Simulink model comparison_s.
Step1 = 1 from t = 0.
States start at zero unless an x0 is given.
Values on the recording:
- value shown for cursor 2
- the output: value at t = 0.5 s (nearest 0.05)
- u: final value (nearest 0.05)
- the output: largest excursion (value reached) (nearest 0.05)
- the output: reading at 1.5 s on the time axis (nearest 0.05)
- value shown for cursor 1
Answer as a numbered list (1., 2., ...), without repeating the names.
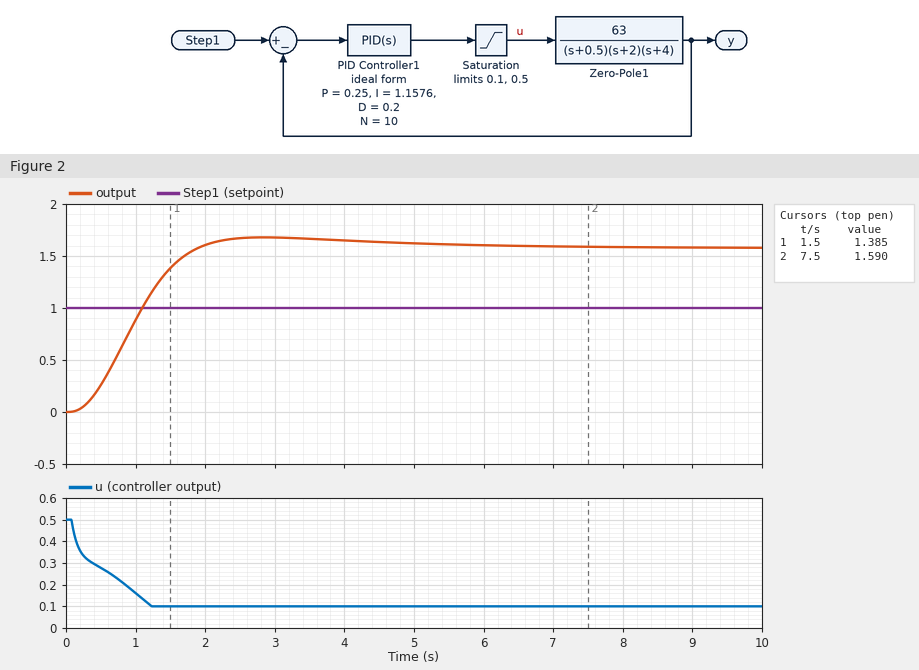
1. 1.590
2. 0.25
3. 0.10
4. 1.70
5. 1.40
6. 1.385
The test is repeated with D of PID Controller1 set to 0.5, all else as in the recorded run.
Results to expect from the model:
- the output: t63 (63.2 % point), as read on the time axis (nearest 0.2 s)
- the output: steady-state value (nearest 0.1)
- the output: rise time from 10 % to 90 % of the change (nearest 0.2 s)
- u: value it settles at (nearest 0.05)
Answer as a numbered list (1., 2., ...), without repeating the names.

1. 1.2 s
2. 1.6
3. 1.8 s
4. 0.10
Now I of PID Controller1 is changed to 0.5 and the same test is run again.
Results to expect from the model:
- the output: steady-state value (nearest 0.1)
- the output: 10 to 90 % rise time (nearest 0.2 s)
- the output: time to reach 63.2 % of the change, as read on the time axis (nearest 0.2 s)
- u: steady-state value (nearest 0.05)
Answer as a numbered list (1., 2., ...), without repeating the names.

1. 1.6
2. 2.2 s
3. 1.2 s
4. 0.10
